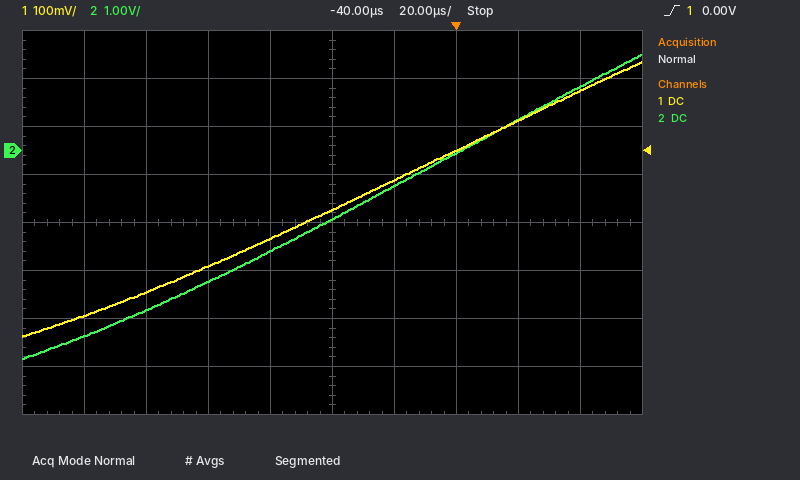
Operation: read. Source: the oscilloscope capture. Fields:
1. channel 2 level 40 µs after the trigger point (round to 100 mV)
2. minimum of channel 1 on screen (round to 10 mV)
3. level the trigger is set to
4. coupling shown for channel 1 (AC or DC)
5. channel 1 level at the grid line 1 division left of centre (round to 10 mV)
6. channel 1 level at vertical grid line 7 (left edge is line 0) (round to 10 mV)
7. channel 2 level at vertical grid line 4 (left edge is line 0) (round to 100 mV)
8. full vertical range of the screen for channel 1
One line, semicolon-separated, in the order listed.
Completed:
1.3 V; -390 mV; 0.00 V; DC; -180 mV; 0 mV; -2.1 V; 800 mV
